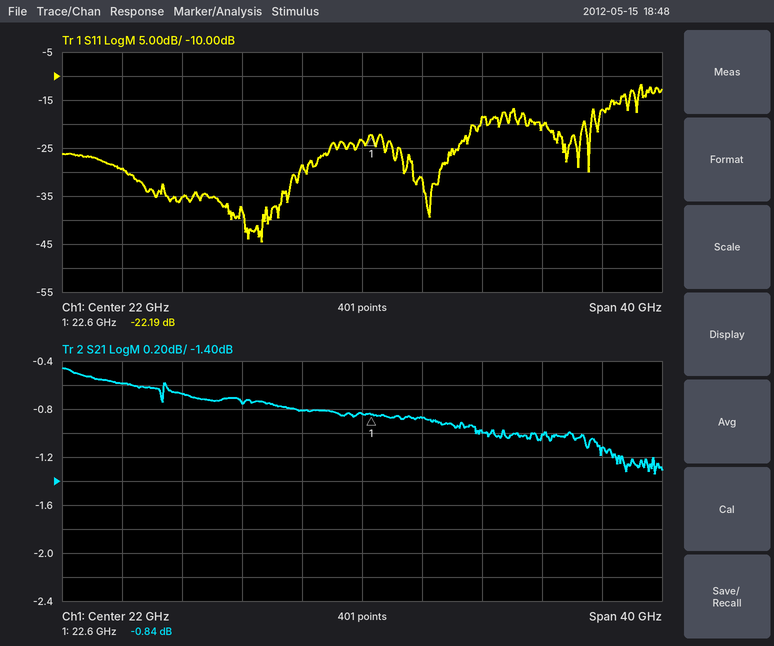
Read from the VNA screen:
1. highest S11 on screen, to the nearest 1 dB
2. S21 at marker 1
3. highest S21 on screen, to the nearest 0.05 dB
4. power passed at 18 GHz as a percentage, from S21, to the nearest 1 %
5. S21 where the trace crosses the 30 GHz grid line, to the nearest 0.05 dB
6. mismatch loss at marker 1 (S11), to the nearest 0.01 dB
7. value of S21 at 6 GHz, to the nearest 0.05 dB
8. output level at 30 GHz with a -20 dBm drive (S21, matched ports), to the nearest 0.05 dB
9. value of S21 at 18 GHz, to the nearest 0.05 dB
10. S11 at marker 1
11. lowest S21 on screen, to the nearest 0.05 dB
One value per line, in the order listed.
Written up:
-12 dB
-0.84 dB
-0.45 dB
83 %
-1.00 dB
0.03 dB
-0.60 dB
-21.00 dBm
-0.80 dB
-22.19 dB
-1.35 dB
